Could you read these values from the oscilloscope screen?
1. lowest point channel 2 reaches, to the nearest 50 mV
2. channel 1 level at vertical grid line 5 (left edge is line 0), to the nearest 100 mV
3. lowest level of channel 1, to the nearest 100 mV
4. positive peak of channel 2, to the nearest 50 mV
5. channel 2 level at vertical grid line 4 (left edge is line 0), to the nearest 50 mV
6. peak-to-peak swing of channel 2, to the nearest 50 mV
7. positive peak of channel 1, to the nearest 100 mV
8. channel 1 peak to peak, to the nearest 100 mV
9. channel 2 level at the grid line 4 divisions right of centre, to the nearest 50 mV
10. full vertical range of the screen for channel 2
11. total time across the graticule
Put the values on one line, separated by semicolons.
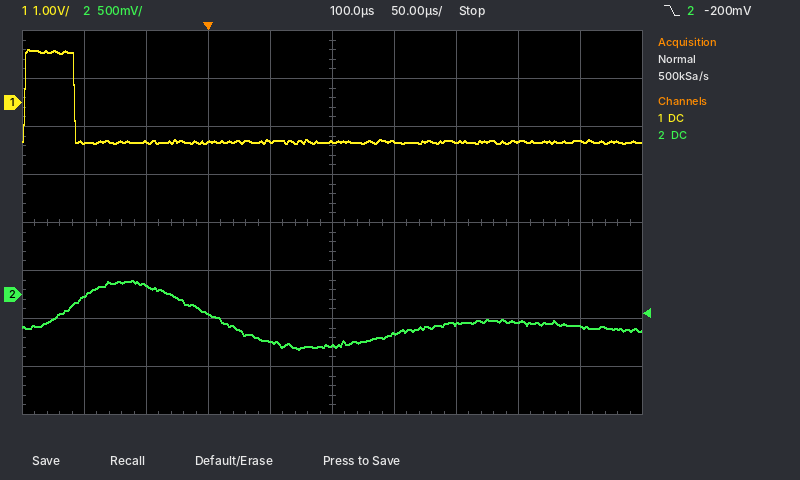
-550 mV; -800 mV; -900 mV; 150 mV; -500 mV; 700 mV; 1.1 V; 2.0 V; -350 mV; 4 V; 500 µs
